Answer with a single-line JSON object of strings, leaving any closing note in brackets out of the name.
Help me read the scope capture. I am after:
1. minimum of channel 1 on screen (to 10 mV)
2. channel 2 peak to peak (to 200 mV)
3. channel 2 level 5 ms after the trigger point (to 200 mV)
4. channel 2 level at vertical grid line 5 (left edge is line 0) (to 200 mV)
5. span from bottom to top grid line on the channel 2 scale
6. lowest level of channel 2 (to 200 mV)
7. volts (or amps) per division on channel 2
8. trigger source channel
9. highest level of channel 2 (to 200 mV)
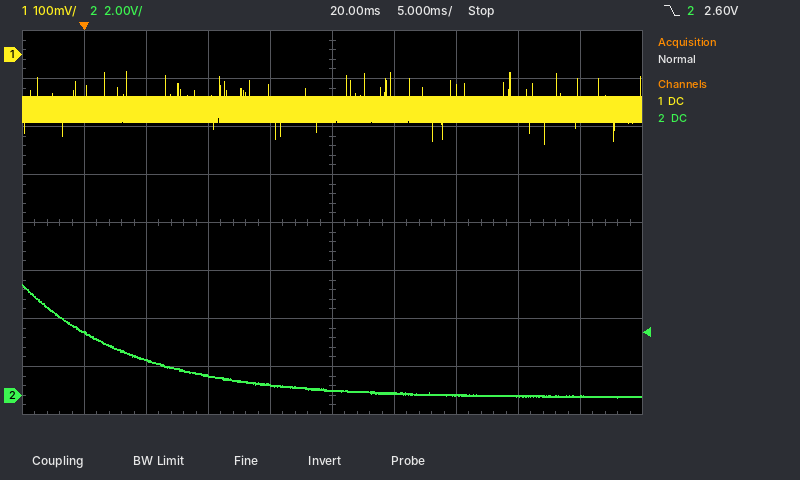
{"minimum of channel 1 on screen": "-190 mV", "channel 2 peak to peak": "4.8 V", "channel 2 level 5 ms after the trigger point": "1.4 V", "channel 2 level at vertical grid line 5 (left edge is line 0)": "200 mV", "span from bottom to top grid line on the channel 2 scale": "16 V", "lowest level of channel 2": "-200 mV", "volts (or amps) per division on channel 2": "2 V", "trigger source channel": "channel 2", "highest level of channel 2": "4.6 V"}
